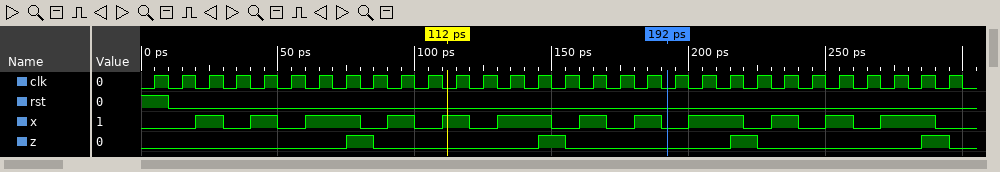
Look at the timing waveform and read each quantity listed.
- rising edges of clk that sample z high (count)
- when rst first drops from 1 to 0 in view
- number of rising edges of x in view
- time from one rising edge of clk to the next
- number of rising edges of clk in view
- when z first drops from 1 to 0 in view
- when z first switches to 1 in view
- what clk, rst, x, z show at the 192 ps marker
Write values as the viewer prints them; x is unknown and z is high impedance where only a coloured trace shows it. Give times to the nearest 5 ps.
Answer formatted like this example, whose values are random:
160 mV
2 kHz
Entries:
4
10 ps
12
10 ps
30
85 ps
75 ps
clk=0, rst=0, x=0, z=0
